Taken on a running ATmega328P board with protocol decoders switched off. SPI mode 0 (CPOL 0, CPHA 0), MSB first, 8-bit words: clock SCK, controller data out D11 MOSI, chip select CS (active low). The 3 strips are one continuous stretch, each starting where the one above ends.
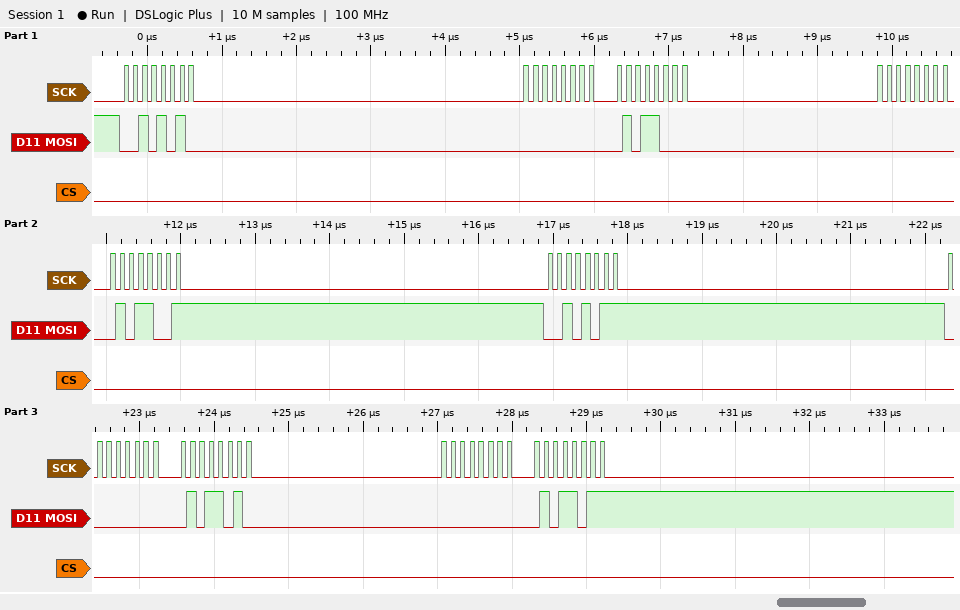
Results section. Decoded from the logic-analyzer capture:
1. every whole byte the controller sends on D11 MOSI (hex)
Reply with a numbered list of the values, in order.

1. 2A 00 58 00 59 2B 00 5A 00 5B
